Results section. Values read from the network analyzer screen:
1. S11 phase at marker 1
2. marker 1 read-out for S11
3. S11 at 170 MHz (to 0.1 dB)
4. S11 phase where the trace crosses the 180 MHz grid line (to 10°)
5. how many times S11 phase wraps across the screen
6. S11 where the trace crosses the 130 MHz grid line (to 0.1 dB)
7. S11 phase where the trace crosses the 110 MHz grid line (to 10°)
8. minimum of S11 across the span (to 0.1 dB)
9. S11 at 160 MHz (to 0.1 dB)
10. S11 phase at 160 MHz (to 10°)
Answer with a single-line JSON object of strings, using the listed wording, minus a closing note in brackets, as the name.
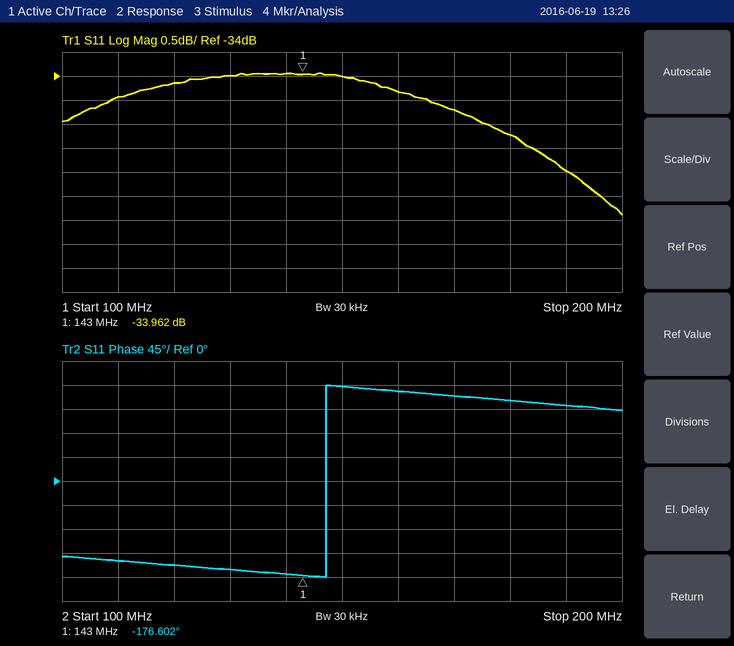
{"S11 phase at marker 1": "-176.602°", "marker 1 read-out for S11": "-33.962 dB", "S11 at 170 MHz": "-34.7 dB", "S11 phase where the trace crosses the 180 MHz grid line": "150°", "how many times S11 phase wraps across the screen": "1", "S11 where the trace crosses the 130 MHz grid line": "-34.0 dB", "S11 phase where the trace crosses the 110 MHz grid line": "-150°", "minimum of S11 across the span": "-36.9 dB", "S11 at 160 MHz": "-34.3 dB", "S11 phase at 160 MHz": "170°"}
